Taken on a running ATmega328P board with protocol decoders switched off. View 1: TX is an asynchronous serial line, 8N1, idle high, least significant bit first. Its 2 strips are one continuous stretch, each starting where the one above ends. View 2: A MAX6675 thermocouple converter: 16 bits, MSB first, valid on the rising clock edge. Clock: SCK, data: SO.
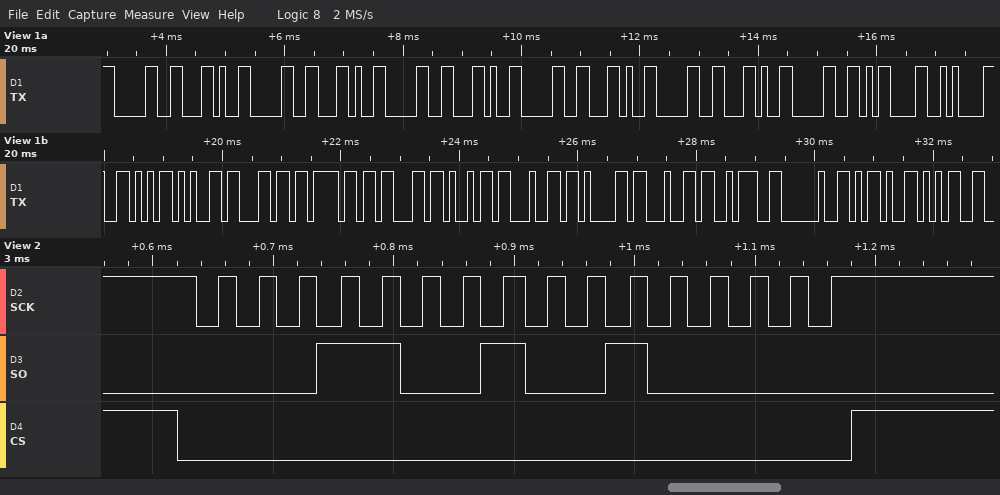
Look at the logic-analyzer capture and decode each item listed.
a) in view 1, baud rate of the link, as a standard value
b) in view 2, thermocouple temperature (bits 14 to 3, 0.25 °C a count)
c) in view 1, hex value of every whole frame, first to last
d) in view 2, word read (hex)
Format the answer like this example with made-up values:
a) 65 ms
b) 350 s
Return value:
a) 9600 baud
b) 201.00 °C
c) 30 2C 30 2C 30 2C 30 2C 30 2C 30 0D 0A 56 65 6C 6F 63 69 64 61 64 3A 20 2D 35
d) 0x1920
